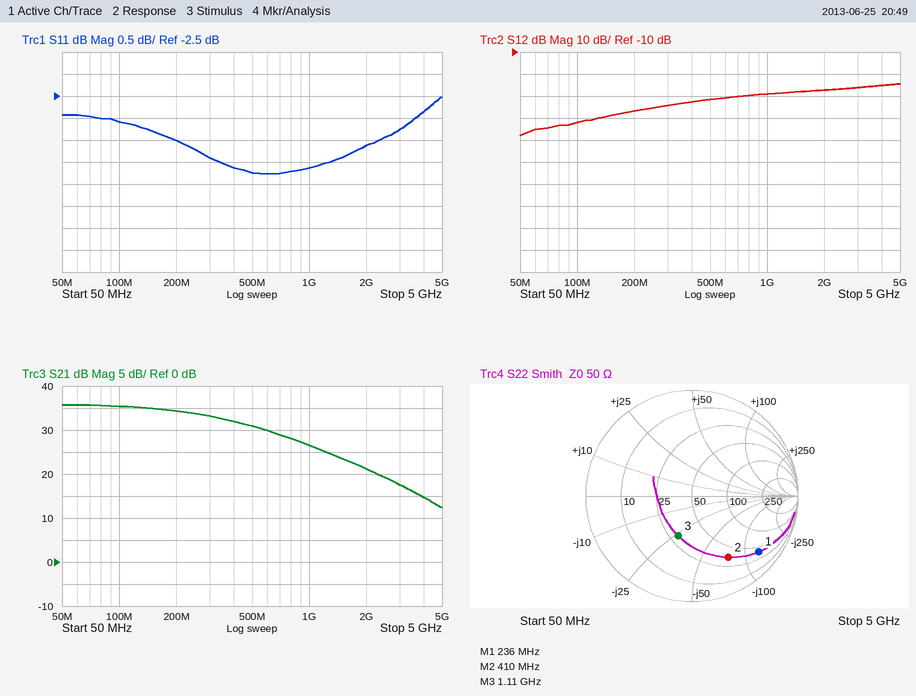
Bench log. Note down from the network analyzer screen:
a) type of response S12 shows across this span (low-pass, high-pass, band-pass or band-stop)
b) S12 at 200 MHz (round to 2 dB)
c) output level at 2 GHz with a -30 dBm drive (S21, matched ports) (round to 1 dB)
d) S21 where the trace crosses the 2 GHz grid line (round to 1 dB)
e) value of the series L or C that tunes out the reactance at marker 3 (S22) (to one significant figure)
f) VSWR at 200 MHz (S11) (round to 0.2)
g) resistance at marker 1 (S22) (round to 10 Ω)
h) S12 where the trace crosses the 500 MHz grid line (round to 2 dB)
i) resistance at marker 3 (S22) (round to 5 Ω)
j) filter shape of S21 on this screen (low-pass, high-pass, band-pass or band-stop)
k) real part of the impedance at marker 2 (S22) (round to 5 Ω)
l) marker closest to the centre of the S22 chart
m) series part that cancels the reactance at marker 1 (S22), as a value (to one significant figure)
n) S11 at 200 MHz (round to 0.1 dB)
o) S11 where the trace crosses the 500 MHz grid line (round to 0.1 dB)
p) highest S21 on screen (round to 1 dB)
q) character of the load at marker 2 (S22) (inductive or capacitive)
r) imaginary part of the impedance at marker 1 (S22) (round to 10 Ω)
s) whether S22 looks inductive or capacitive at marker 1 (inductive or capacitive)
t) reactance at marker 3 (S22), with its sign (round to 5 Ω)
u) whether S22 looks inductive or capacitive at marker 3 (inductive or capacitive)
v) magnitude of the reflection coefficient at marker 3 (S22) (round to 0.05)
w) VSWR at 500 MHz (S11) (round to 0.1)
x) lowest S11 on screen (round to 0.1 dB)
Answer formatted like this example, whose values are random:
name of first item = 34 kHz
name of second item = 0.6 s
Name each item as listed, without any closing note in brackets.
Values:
type of response S12 shows across this span = high-pass
S12 at 200 MHz = -36 dB
output level at 2 GHz with a -30 dBm drive (S21, matched ports) = -9 dBm
S21 where the trace crosses the 2 GHz grid line = 21 dB
value of the series L or C that tunes out the reactance at marker 3 (S22) = 4 nH
VSWR at 200 MHz (S11) = 5.0
resistance at marker 1 (S22) = 40 Ω
S12 where the trace crosses the 500 MHz grid line = -32 dB
resistance at marker 3 (S22) = 30 Ω
filter shape of S21 on this screen = low-pass
real part of the impedance at marker 2 (S22) = 35 Ω
marker closest to the centre of the S22 chart = marker 3
series part that cancels the reactance at marker 1 (S22), as a value = 90 nH
S11 at 200 MHz = -3.5 dB
S11 where the trace crosses the 500 MHz grid line = -4.2 dB
highest S21 on screen = 36 dB
character of the load at marker 2 (S22) = capacitive
imaginary part of the impedance at marker 1 (S22) = -130 Ω
whether S22 looks inductive or capacitive at marker 1 = capacitive
reactance at marker 3 (S22), with its sign = -25 Ω
whether S22 looks inductive or capacitive at marker 3 = capacitive
magnitude of the reflection coefficient at marker 3 (S22) = 0.40
VSWR at 500 MHz (S11) = 4.2
lowest S11 on screen = -4.3 dB
